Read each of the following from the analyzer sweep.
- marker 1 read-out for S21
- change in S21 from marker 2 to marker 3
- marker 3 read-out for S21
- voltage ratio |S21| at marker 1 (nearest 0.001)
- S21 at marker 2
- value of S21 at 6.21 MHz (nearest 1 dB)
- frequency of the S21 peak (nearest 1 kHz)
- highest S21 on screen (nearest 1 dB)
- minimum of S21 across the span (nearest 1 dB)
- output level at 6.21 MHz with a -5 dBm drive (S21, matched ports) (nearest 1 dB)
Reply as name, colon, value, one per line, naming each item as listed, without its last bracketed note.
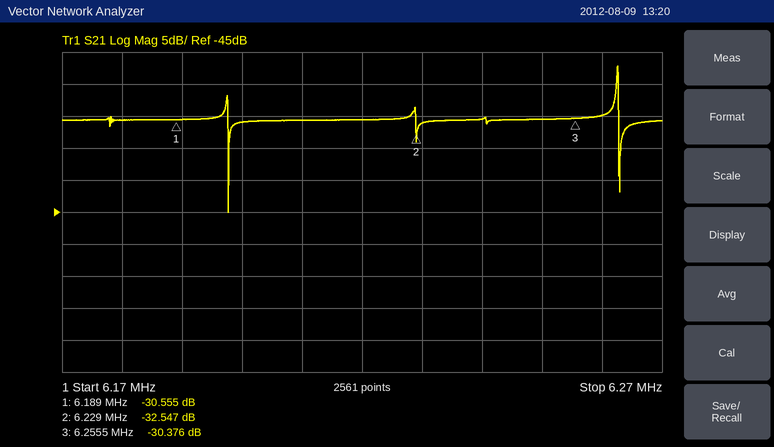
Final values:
marker 1 read-out for S21: -30.555 dB
change in S21 from marker 2 to marker 3: 2.171 dB
marker 3 read-out for S21: -30.376 dB
voltage ratio |S21| at marker 1: 0.030
S21 at marker 2: -32.547 dB
value of S21 at 6.21 MHz: -31 dB
frequency of the S21 peak: 6.263 MHz
highest S21 on screen: -22 dB
minimum of S21 across the span: -45 dB
output level at 6.21 MHz with a -5 dBm drive (S21, matched ports): -36 dBm
